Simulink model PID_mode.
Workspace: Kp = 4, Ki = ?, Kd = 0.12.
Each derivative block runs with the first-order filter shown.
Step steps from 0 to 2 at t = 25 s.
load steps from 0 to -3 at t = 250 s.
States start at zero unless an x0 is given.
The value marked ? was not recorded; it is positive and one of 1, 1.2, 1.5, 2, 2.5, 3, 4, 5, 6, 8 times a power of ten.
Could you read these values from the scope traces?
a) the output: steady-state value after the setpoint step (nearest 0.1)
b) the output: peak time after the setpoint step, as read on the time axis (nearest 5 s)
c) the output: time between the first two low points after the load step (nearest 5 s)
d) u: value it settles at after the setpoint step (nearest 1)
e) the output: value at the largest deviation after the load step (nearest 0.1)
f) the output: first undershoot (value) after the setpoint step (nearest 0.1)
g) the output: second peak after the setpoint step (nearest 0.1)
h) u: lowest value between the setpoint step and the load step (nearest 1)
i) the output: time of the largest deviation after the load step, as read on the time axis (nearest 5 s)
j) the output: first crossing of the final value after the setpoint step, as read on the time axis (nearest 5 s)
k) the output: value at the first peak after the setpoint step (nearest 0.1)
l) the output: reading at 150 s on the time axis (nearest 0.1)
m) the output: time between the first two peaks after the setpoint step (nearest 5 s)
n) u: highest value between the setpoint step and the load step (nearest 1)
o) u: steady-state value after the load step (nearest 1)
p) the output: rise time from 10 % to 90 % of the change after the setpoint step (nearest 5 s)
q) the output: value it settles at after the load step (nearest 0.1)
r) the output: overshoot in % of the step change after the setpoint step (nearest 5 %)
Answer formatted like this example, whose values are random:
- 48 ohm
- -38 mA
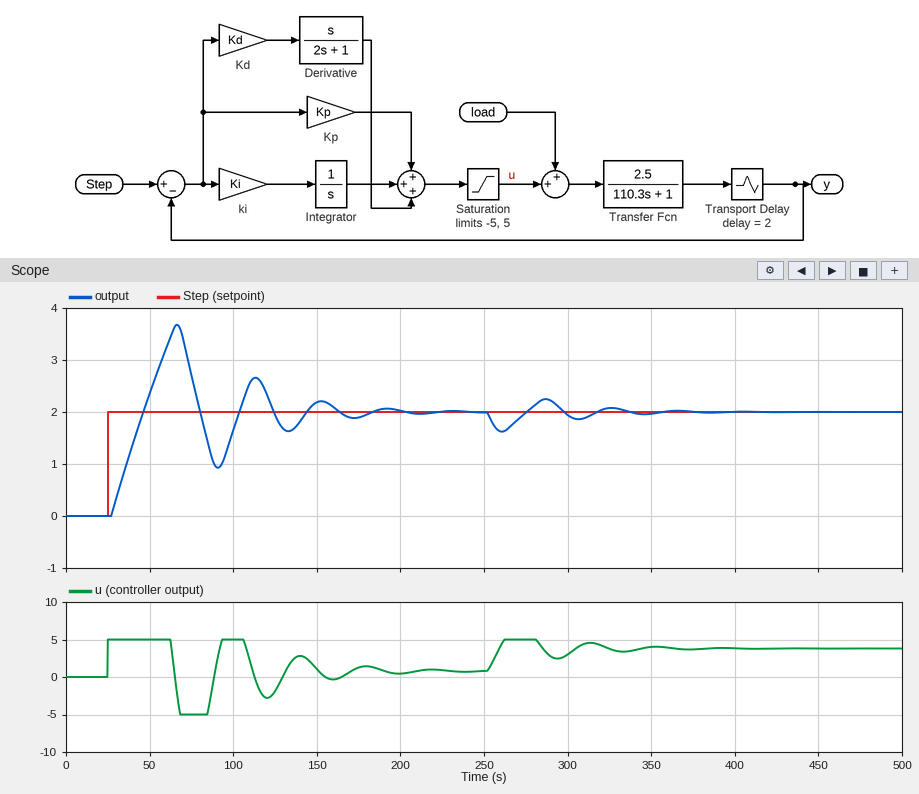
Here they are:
- 2.0
- 65 s
- 45 s
- 1
- 1.6
- 0.9
- 2.7
- -5
- 260 s
- 45 s
- 3.7
- 2.2
- 45 s
- 5
- 4
- 15 s
- 2.0
- 85 %
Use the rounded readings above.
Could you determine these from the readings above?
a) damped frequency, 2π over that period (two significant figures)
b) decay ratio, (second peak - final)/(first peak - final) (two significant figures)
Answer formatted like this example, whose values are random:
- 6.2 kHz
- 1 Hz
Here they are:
- 0.14 rad/s
- 0.41
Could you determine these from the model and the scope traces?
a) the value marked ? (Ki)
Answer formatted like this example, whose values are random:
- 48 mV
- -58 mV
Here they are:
- 1
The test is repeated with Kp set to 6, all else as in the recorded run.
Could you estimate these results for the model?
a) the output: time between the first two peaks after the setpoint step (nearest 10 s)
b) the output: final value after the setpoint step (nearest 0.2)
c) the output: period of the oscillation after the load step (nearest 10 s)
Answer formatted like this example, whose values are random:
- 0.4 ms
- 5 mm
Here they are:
- 40 s
- 2.0
- 40 s
